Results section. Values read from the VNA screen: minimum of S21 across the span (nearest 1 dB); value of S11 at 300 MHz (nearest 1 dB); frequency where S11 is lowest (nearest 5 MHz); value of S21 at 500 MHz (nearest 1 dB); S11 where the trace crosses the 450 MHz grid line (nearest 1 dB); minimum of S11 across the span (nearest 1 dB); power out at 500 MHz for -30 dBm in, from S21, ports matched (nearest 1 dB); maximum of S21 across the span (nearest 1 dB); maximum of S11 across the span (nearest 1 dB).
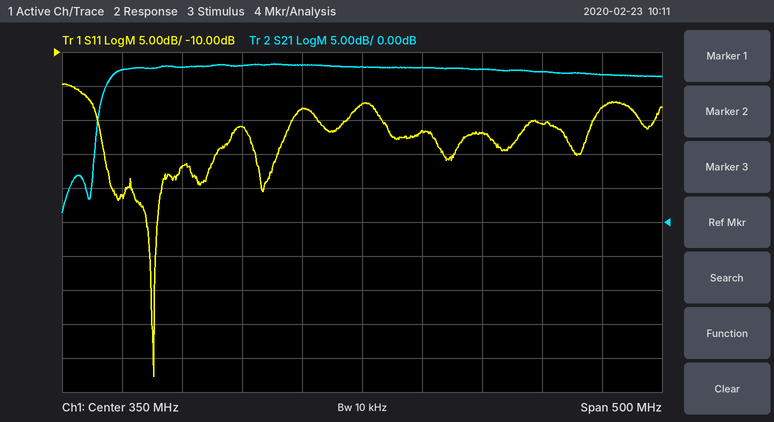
1 dB
-18 dB
175 MHz
22 dB
-22 dB
-58 dB
-8 dBm
23 dB
-15 dB
